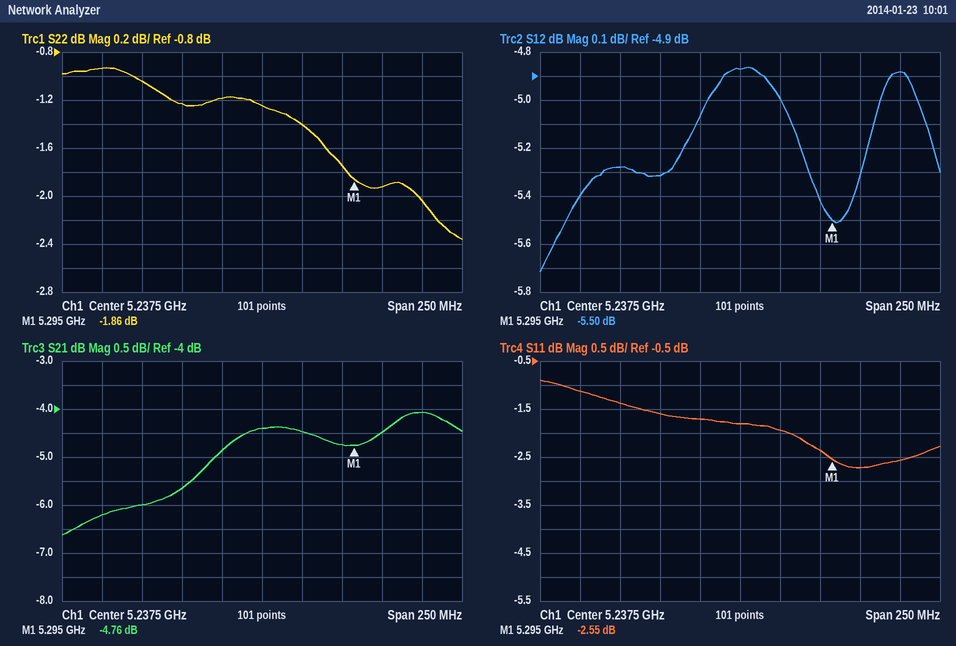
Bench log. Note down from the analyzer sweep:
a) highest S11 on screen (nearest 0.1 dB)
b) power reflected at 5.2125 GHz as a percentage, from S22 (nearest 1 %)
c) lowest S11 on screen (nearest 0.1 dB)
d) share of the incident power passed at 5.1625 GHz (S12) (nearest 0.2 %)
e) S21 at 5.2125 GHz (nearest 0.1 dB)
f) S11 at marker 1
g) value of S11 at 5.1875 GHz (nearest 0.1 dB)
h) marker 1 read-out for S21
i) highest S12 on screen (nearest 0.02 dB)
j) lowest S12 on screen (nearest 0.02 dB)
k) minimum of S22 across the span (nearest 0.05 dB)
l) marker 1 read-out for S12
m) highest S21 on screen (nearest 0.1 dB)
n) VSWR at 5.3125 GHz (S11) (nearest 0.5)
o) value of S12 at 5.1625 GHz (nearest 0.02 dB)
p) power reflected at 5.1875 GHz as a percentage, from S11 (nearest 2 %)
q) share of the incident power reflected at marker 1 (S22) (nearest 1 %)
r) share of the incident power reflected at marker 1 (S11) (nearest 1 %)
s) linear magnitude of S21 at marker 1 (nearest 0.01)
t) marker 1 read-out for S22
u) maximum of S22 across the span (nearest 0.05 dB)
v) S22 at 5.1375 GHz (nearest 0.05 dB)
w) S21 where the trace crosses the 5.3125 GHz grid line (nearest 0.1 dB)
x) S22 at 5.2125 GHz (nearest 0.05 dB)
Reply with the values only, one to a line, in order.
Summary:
-0.9 dB
76 %
-2.7 dB
29.6 %
-4.9 dB
-2.55 dB
-1.6 dB
-4.76 dB
-4.86 dB
-5.72 dB
-2.35 dB
-5.50 dB
-4.1 dB
6.5
-5.28 dB
70 %
65 %
56 %
0.58
-1.86 dB
-0.95 dB
-0.95 dB
-4.5 dB
-1.20 dB
